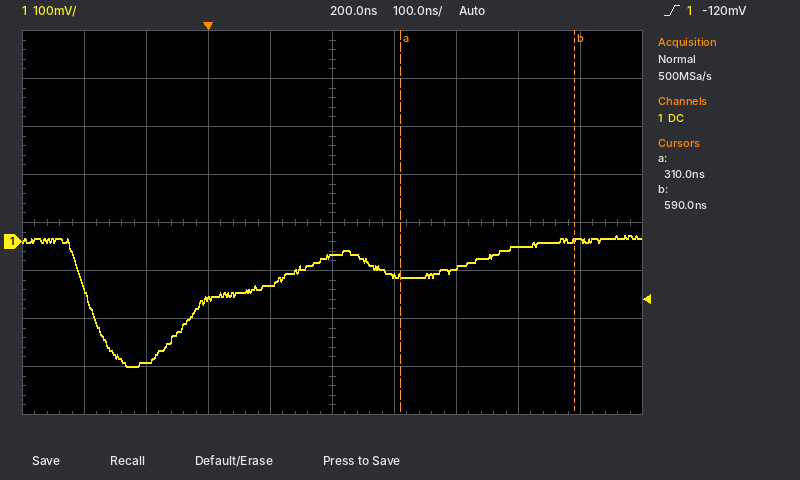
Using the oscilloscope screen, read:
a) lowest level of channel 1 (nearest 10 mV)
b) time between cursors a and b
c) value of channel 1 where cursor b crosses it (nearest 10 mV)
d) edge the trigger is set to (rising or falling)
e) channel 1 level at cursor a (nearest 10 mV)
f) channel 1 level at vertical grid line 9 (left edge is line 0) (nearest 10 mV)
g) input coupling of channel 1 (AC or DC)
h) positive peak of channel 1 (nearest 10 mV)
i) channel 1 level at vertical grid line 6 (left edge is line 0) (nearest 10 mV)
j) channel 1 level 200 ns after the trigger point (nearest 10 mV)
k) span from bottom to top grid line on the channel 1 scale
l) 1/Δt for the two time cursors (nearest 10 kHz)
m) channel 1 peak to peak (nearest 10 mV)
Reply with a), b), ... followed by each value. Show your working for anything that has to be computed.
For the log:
a) -260 mV
b) 590 ns − (310 ns) = 280 ns
c) 0 mV
d) rising
e) -70 mV
f) 0 mV
g) DC
h) 10 mV
i) -70 mV
j) -30 mV
k) 800 mV
l) 1 / 280 ns ≈ 3.57 MHz
m) 10 mV − (-260 mV) = 270 mV
